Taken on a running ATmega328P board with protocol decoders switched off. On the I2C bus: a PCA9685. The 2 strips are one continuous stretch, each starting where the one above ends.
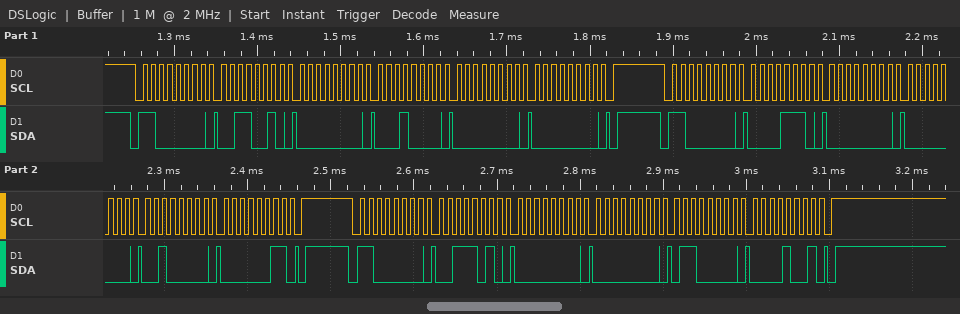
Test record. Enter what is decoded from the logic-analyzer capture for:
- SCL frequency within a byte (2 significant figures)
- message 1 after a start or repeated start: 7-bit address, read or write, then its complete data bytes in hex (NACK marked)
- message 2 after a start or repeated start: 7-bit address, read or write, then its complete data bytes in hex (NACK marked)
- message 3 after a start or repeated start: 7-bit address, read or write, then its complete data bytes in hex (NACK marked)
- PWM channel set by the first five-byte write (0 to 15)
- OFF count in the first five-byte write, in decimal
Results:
100 kHz
0x60 write: 32 00 10 00 00
0x60 write: 0E 00 00 20 03
0x60 write: 3A 00 00 60 09
11
0
